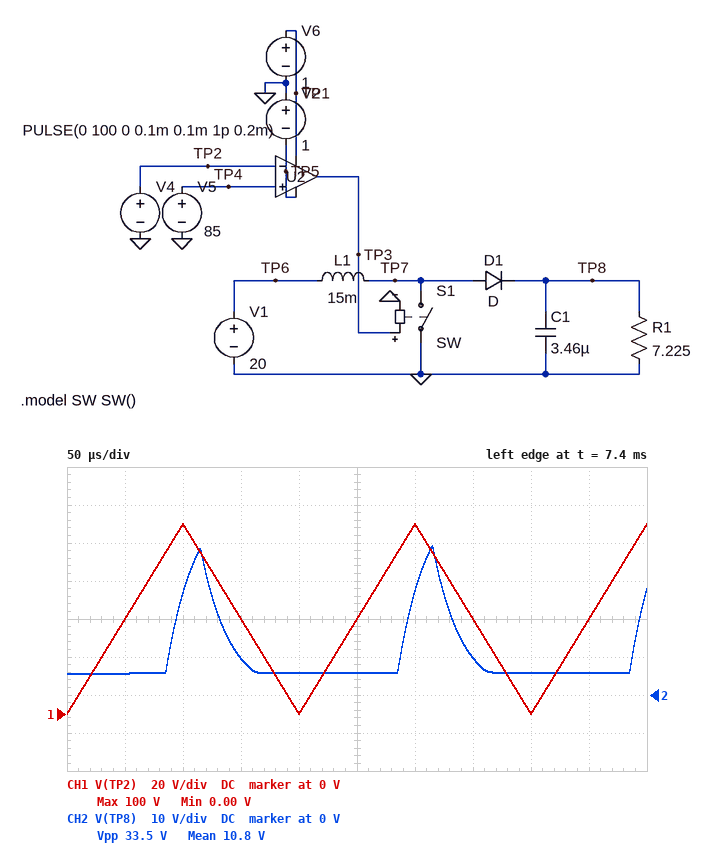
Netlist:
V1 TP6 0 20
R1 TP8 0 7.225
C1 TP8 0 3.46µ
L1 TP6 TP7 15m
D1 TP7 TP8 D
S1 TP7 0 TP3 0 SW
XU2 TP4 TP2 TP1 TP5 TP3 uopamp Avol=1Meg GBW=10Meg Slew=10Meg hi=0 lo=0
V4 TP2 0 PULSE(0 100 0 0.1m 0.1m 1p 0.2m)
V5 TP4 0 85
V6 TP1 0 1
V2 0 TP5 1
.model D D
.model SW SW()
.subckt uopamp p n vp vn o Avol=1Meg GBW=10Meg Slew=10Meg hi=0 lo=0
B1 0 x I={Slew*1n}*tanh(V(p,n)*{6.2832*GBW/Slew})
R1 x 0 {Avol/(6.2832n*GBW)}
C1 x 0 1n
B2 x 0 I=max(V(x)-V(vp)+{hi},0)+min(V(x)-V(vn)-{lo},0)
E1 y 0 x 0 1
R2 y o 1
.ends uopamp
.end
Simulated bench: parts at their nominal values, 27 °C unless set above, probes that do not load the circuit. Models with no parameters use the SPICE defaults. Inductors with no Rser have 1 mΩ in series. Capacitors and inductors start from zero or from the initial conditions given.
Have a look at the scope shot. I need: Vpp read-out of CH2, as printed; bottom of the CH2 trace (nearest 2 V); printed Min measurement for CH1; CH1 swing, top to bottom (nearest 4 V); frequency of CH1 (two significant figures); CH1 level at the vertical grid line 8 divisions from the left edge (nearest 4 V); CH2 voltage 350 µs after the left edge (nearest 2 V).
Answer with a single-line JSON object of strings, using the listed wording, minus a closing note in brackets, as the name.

{"Vpp read-out of CH2, as printed": "33.5 V", "bottom of the CH2 trace": "6 V", "printed Min measurement for CH1": "0.00 V", "CH1 swing, top to bottom": "100 V", "frequency of CH1": "5.0 kHz", "CH1 level at the vertical grid line 8 divisions from the left edge": "0 V", "CH2 voltage 350 µs after the left edge": "10 V"}
